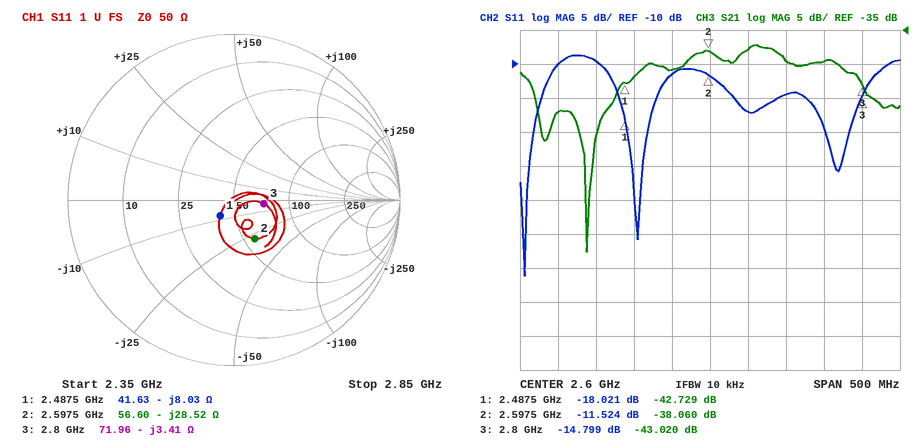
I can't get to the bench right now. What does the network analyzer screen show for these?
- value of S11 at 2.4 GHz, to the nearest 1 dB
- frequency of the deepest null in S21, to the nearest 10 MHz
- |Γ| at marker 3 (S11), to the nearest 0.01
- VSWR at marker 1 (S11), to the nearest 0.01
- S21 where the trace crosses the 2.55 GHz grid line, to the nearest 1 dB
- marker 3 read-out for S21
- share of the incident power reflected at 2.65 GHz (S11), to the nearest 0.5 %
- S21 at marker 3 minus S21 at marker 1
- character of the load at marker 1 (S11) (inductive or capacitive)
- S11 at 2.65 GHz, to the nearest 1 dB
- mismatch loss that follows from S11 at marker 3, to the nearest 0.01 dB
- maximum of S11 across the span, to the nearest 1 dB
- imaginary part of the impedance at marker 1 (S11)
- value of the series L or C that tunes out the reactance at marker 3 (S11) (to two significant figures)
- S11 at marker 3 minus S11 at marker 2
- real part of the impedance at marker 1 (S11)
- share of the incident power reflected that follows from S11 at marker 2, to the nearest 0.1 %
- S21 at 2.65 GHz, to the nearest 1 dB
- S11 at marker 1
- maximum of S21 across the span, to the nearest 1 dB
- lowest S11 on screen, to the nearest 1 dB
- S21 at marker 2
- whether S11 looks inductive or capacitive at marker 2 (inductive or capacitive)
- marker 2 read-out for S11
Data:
-10 dB
2.44 GHz
0.18
1.29
-41 dB
-43.020 dB
2.0 %
-0.291 dB
capacitive
-17 dB
0.15 dB
-9 dB
-8.03 Ω
190 pH
-3.275 dB
41.63 Ω
7.0 %
-38 dB
-18.021 dB
-37 dB
-41 dB
-38.060 dB
capacitive
-11.524 dB
